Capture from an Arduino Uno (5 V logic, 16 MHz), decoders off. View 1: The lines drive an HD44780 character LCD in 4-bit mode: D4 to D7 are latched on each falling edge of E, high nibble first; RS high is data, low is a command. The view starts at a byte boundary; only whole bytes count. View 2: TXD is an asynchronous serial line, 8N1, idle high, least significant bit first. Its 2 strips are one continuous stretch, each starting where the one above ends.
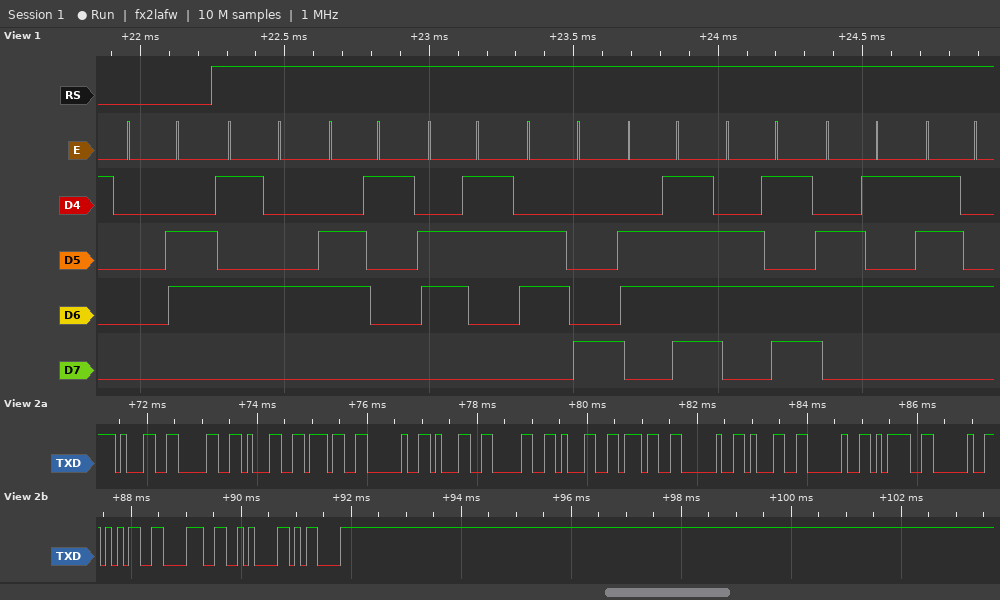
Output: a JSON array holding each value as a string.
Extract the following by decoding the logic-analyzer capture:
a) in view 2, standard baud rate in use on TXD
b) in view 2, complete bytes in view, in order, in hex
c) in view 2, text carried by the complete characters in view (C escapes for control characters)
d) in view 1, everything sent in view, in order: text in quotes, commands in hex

["9600 baud", "0x31 0x30 0x31 0x37 0x20 0x31 0x30 0x31 0x37 0x20 0x31 0x20 0x3D 0x20 0x35 0x38 0x0A 0x0D", "\"1017 1017 1 = 58\\n\\r\"", "0x06 \"Tachomet\""]
